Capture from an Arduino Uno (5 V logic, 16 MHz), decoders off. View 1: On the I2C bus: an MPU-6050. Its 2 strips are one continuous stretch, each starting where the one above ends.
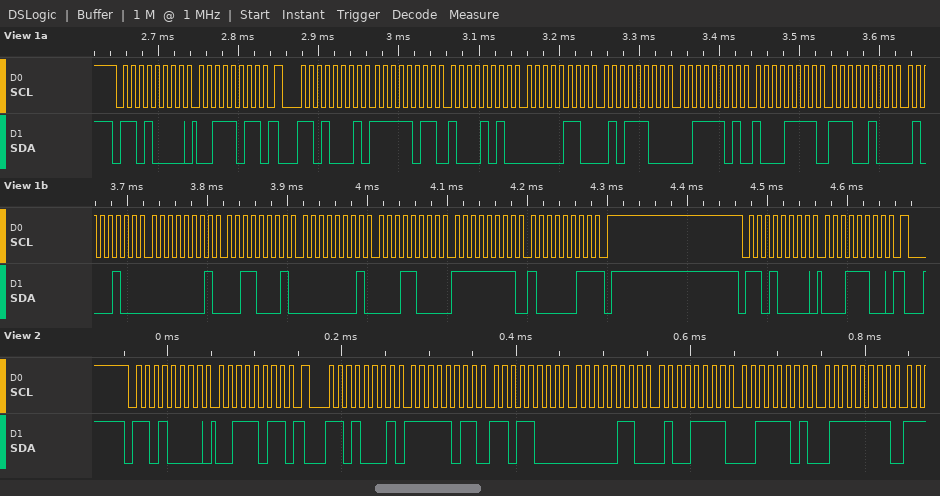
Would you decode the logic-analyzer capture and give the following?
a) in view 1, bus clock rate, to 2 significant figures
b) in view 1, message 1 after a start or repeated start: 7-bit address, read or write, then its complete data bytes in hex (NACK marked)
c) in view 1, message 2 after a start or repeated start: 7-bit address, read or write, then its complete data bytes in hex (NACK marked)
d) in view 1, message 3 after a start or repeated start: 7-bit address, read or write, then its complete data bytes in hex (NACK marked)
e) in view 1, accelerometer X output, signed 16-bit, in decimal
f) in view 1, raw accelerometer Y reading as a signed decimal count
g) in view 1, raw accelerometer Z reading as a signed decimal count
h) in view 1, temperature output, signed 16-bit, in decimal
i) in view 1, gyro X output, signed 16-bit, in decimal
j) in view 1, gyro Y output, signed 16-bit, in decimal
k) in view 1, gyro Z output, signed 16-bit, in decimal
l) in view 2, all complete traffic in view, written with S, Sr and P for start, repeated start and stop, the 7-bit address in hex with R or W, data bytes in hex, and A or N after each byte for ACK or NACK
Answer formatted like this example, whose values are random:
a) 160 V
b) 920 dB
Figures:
a) 100 kHz
b) 0x68 write: 3B
c) 0x68 read: FB 8A 06 5C 3D 8F E4 44 01 31 01 18 FF 83 NACK
d) 0x68 write: 1C
e) -1142
f) 1628
g) 15759
h) -7100
i) 305
j) 280
k) -125
l) S 68W A 3B A Sr 68R A FB A D8 A 06 A 4F A 3D A 7F A
